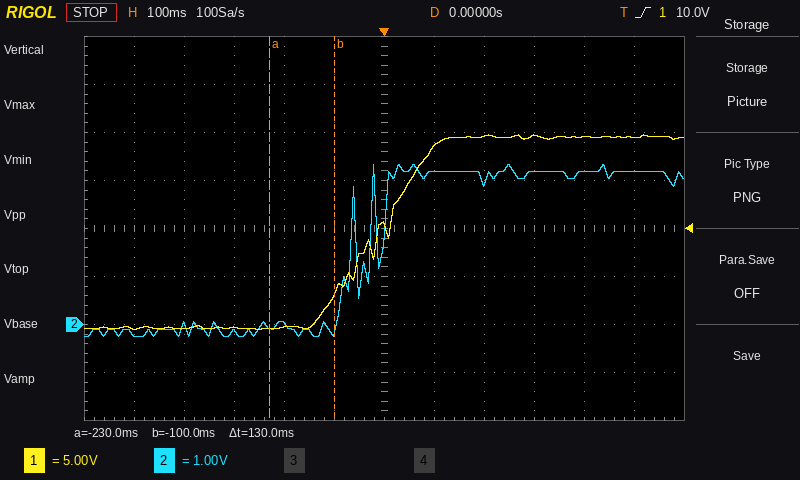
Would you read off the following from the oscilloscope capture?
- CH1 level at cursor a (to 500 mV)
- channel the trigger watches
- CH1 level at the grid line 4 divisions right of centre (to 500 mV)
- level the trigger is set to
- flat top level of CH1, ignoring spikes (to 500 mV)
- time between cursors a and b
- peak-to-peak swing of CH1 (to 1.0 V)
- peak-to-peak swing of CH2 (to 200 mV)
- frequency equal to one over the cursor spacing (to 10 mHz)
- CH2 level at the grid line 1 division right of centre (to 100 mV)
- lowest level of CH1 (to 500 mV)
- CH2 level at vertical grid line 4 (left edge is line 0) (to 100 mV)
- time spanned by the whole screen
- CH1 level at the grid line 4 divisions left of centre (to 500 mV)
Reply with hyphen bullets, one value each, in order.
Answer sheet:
- -500 mV
- CH1
- 19.5 V
- 10.0 V
- 19.5 V
- 130 ms
- 20.0 V
- 3.6 V
- 7.69 Hz
- 3.2 V
- -500 mV
- 0.0 V
- 1.2 s
- -500 mV
